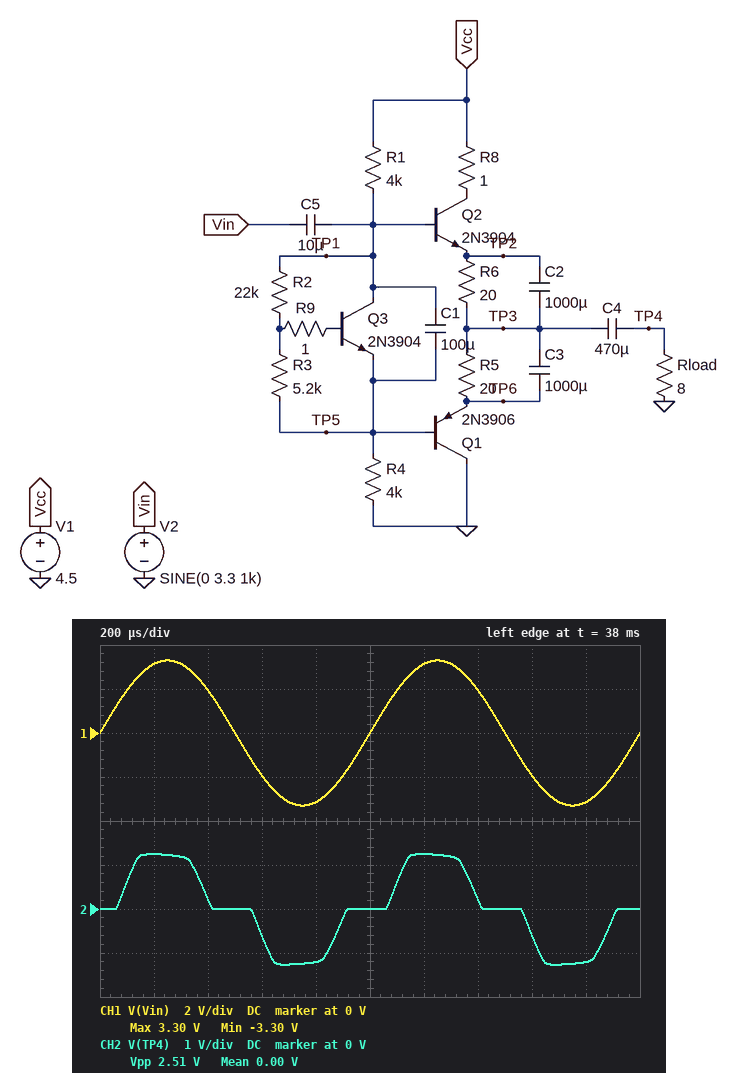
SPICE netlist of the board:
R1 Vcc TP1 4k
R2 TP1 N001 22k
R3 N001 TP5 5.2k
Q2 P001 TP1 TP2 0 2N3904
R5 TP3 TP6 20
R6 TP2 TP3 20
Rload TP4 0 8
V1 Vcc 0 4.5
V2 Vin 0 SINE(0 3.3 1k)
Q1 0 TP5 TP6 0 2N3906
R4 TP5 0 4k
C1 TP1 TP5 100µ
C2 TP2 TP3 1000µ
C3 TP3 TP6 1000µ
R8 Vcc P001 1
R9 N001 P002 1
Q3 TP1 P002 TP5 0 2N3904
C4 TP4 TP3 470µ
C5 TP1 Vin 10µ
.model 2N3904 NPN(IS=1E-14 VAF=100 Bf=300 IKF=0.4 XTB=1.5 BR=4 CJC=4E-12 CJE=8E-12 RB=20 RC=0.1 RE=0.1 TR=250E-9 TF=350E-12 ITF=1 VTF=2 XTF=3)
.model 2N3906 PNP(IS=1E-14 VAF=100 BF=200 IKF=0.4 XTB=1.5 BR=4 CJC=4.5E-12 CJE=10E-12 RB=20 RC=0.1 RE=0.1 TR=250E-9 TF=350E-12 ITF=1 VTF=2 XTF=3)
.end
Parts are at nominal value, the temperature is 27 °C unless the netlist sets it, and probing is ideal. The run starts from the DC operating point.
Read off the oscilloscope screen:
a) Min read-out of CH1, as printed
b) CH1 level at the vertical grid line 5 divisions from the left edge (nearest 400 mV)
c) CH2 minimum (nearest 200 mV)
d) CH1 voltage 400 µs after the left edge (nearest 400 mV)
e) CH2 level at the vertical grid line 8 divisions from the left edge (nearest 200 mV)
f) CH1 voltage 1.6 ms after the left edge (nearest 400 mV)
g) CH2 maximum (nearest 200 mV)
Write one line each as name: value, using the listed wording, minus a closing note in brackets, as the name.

Min read-out of CH1, as printed: -3.30 V
CH1 level at the vertical grid line 5 divisions from the left edge: 0 V
CH2 minimum: -1.2 V
CH1 voltage 400 µs after the left edge: 2.0 V
CH2 level at the vertical grid line 8 divisions from the left edge: -600 mV
CH1 voltage 1.6 ms after the left edge: -2.0 V
CH2 maximum: 1.2 V
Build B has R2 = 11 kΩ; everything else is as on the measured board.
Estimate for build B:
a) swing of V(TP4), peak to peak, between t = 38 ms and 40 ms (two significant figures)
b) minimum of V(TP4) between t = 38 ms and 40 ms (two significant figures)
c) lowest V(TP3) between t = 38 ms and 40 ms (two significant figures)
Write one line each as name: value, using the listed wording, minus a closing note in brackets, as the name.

swing of V(TP4), peak to peak, between t = 38 ms and 40 ms: 2.6 V
minimum of V(TP4) between t = 38 ms and 40 ms: -1.3 V
lowest V(TP3) between t = 38 ms and 40 ms: 920 mV
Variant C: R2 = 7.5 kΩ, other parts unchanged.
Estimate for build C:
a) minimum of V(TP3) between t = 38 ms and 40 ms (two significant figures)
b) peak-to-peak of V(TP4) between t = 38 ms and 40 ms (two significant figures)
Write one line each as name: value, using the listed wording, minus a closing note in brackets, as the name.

minimum of V(TP3) between t = 38 ms and 40 ms: 900 mV
peak-to-peak of V(TP4) between t = 38 ms and 40 ms: 2.6 V
